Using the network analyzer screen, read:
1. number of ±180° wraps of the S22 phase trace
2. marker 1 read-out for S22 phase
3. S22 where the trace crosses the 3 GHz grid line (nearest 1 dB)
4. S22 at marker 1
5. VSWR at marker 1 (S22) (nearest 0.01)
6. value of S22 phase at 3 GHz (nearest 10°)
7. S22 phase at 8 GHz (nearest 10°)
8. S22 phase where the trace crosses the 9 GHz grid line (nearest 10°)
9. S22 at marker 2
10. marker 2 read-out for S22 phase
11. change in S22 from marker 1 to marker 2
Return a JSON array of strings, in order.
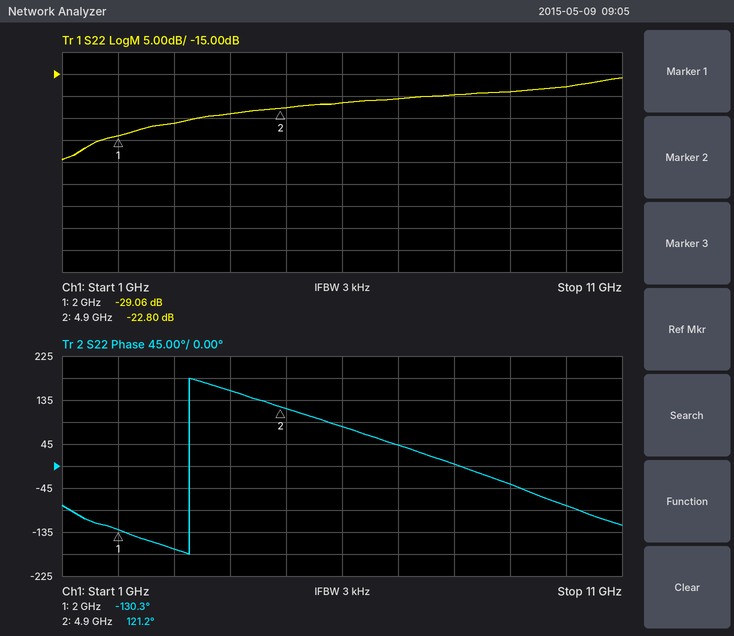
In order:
["1", "-130.3°", "-26 dB", "-29.06 dB", "1.07", "-170°", "0°", "-40°", "-22.80 dB", "121.2°", "6.26 dB"]
